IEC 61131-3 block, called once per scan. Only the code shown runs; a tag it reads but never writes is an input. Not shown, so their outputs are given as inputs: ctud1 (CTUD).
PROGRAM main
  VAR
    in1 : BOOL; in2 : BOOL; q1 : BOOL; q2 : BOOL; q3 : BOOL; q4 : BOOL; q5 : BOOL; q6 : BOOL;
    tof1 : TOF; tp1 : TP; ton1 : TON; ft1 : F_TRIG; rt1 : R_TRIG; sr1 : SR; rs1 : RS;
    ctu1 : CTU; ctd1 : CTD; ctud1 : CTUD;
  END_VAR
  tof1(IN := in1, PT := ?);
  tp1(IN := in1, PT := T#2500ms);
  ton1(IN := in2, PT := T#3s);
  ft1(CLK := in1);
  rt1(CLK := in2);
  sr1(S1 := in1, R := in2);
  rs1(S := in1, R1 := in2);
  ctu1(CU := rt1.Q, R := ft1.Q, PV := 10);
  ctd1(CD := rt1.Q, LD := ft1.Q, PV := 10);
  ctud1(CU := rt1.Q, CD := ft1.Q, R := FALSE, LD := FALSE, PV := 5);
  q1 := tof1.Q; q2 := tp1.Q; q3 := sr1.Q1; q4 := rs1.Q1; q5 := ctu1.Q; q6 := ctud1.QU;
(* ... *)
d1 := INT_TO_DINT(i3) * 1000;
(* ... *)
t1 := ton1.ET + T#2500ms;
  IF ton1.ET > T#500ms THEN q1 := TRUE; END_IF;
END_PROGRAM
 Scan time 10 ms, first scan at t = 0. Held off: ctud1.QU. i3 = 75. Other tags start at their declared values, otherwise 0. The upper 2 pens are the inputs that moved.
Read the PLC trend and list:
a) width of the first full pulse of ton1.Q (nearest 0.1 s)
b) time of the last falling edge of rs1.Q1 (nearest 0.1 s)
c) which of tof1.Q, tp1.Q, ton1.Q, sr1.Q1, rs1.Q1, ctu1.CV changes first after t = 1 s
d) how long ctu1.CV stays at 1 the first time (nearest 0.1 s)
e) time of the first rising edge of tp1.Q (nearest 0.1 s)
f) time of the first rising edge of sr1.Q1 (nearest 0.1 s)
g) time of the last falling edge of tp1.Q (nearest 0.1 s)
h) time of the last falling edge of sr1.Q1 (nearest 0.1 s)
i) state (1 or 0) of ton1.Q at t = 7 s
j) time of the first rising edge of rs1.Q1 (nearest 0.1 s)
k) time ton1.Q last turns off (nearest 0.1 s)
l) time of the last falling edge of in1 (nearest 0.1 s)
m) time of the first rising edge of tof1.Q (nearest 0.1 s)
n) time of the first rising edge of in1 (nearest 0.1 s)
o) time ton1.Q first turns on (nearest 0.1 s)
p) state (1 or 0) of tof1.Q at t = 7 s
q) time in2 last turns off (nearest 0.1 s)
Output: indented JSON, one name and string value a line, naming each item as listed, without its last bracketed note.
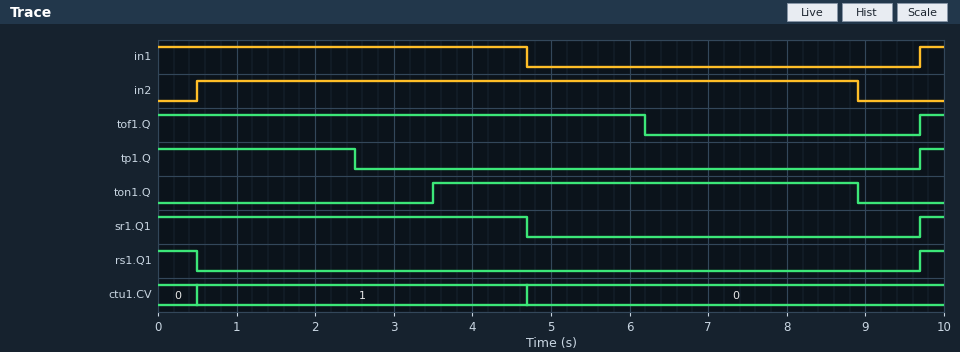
{
  "width of the first full pulse of ton1.Q": "5.4 s",
  "time of the last falling edge of rs1.Q1": "0.5 s",
  "which of tof1.Q, tp1.Q, ton1.Q, sr1.Q1, rs1.Q1, ctu1.CV changes first after t = 1 s": "tp1.Q",
  "how long ctu1.CV stays at 1 the first time": "4.2 s",
  "time of the first rising edge of tp1.Q": "9.7 s",
  "time of the first rising edge of sr1.Q1": "9.7 s",
  "time of the last falling edge of tp1.Q": "2.5 s",
  "time of the last falling edge of sr1.Q1": "4.7 s",
  "state (1 or 0) of ton1.Q at t = 7 s": "1",
  "time of the first rising edge of rs1.Q1": "9.7 s",
  "time ton1.Q last turns off": "8.9 s",
  "time of the last falling edge of in1": "4.7 s",
  "time of the first rising edge of tof1.Q": "9.7 s",
  "time of the first rising edge of in1": "9.7 s",
  "time ton1.Q first turns on": "3.5 s",
  "state (1 or 0) of tof1.Q at t = 7 s": "0",
  "time in2 last turns off": "8.9 s"
}
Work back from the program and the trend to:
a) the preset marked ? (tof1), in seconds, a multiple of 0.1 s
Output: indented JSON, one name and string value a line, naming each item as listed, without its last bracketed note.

{
  "the preset marked ? (tof1), in seconds, a multiple of 0.1 s": "1.5 s"
}
